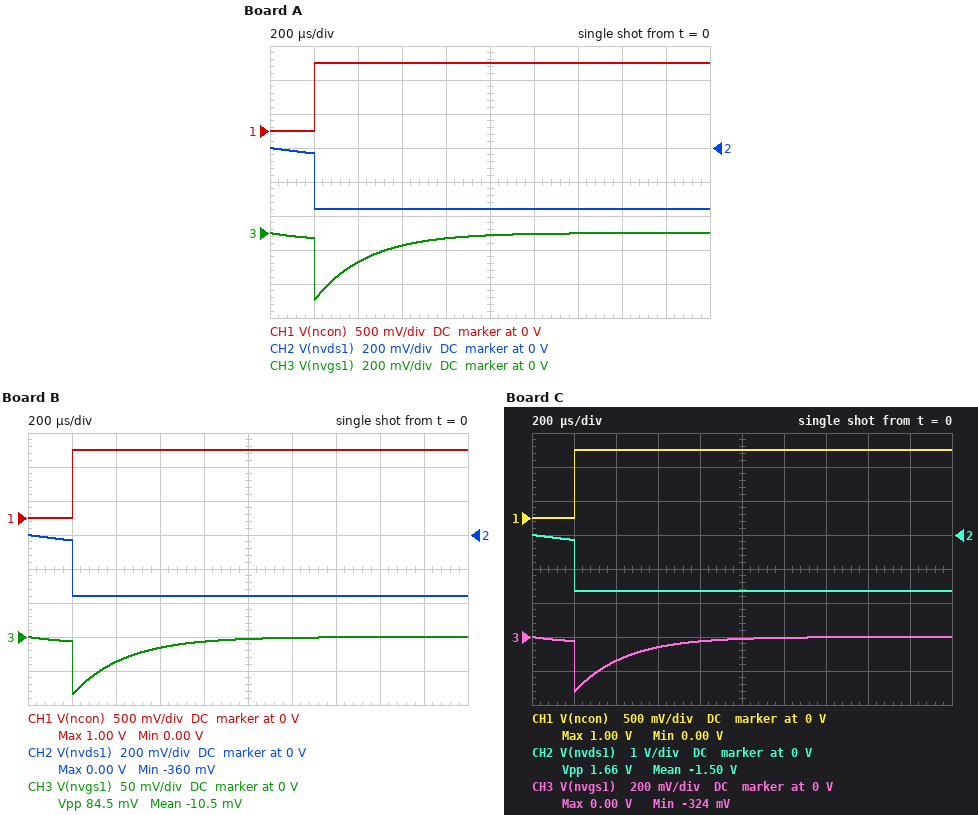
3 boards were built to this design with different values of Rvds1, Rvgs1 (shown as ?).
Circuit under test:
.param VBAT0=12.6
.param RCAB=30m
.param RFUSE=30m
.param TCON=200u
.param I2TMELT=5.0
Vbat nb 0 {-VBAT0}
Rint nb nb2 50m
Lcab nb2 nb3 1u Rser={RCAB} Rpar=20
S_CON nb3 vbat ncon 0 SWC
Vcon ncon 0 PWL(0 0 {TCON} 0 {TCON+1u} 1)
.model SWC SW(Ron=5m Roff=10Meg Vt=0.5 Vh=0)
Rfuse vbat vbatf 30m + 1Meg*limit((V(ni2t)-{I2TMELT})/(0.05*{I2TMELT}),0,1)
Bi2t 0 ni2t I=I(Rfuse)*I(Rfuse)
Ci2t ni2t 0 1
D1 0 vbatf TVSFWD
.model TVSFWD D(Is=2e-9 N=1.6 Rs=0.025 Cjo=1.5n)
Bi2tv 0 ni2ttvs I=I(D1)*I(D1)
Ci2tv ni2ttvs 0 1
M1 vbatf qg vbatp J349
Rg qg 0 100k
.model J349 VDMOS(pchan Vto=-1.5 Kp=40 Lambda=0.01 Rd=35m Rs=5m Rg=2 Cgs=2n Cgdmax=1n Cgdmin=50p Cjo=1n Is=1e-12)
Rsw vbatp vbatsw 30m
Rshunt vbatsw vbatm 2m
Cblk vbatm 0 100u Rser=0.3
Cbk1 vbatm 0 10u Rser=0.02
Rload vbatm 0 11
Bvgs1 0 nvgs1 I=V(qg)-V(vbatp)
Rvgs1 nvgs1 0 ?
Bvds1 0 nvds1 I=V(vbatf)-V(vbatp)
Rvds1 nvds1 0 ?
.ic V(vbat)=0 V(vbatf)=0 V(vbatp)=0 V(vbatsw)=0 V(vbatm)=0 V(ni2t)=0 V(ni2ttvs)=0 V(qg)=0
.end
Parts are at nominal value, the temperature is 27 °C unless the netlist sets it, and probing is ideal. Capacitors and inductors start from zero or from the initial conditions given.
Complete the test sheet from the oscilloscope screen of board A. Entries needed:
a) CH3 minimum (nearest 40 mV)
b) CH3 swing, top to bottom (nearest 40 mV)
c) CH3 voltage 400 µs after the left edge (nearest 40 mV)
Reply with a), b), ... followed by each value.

a) -400 mV
b) 400 mV
c) -160 mV
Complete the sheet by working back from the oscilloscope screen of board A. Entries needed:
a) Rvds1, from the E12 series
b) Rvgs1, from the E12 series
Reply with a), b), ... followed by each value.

a) 0.39 Ω
b) 2.2 Ω
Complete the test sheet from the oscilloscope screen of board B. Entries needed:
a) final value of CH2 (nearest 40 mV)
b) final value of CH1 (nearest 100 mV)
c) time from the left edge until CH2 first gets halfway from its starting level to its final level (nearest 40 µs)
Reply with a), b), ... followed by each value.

a) -360 mV
b) 1.0 V
c) 200 µs
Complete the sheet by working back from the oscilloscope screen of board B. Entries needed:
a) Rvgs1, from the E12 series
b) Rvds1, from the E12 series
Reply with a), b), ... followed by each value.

a) 0.47 Ω
b) 0.39 Ω
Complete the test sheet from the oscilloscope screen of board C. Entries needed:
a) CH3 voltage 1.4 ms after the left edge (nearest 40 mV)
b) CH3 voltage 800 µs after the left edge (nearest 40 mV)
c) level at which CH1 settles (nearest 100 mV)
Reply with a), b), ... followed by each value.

a) 0 V
b) -40 mV
c) 1.0 V
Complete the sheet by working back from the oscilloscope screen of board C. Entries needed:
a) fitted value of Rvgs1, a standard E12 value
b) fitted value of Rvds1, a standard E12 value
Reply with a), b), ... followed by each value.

a) 1.8 Ω
b) 1.8 Ω
